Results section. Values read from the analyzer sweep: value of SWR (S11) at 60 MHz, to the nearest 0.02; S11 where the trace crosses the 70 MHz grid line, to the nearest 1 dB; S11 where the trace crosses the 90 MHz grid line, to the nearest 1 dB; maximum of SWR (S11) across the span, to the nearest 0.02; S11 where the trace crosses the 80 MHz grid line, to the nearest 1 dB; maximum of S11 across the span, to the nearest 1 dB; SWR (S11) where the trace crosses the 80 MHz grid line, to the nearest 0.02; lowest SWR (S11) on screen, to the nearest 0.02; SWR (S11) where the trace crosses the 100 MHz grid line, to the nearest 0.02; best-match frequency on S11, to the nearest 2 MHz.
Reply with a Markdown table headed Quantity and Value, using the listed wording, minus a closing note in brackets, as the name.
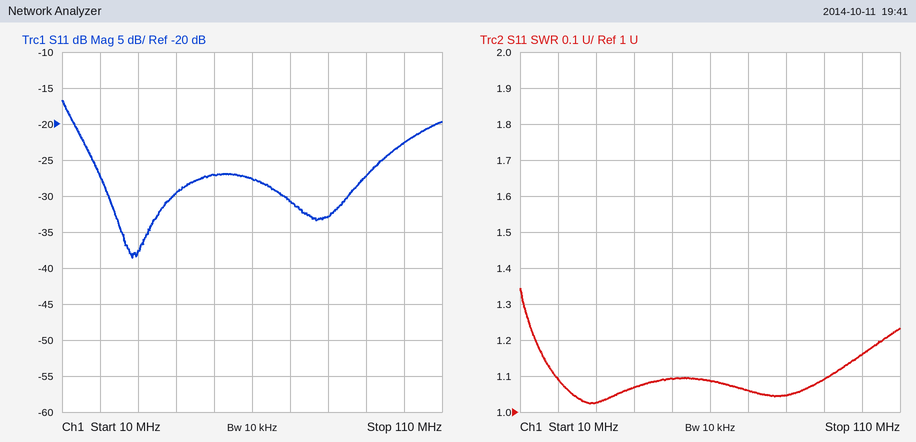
| Quantity | Value |
|---|---|
| value of SWR (S11) at 60 MHz, to the nearest 0.02 | 1.08 |
| S11 where the trace crosses the 70 MHz grid line, to the nearest 1 dB | -31 dB |
| S11 where the trace crosses the 90 MHz grid line, to the nearest 1 dB | -27 dB |
| maximum of SWR (S11) across the span, to the nearest 0.02 | 1.34 |
| S11 where the trace crosses the 80 MHz grid line, to the nearest 1 dB | -33 dB |
| maximum of S11 across the span, to the nearest 1 dB | -17 dB |
| SWR (S11) where the trace crosses the 80 MHz grid line, to the nearest 0.02 | 1.04 |
| lowest SWR (S11) on screen, to the nearest 0.02 | 1.02 |
| SWR (S11) where the trace crosses the 100 MHz grid line, to the nearest 0.02 | 1.16 |
| best-match frequency on S11, to the nearest 2 MHz | 28 MHz |
